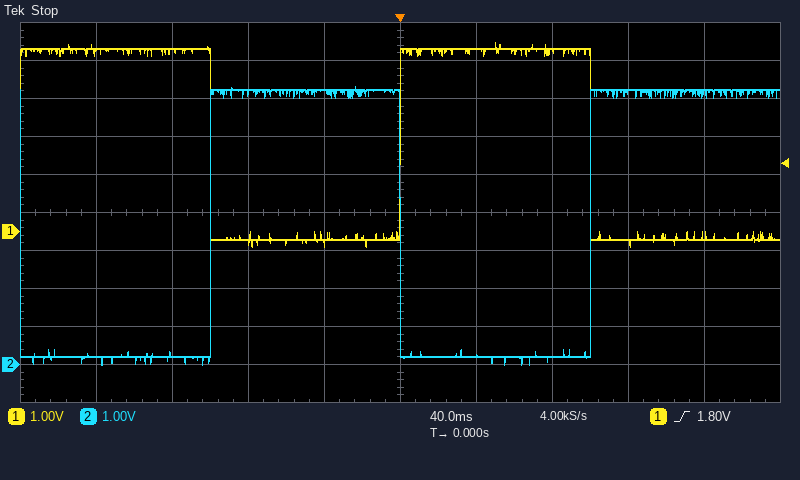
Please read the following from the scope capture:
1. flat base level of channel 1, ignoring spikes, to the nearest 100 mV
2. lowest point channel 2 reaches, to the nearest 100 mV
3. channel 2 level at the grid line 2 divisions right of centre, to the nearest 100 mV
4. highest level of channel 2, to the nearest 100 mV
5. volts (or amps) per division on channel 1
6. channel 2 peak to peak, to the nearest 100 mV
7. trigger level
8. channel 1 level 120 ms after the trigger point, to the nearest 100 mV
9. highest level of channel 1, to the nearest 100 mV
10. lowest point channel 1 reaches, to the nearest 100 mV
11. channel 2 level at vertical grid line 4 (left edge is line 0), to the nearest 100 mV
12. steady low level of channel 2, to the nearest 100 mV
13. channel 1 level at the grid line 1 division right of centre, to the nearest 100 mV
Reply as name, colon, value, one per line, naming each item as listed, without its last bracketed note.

flat base level of channel 1, ignoring spikes, to the nearest 100 mV: -200 mV
lowest point channel 2 reaches, to the nearest 100 mV: 0.0 V
channel 2 level at the grid line 2 divisions right of centre, to the nearest 100 mV: 200 mV
highest level of channel 2, to the nearest 100 mV: 7.3 V
volts (or amps) per division on channel 1: 1 V
channel 2 peak to peak, to the nearest 100 mV: 7.3 V
trigger level: 1.80 V
channel 1 level 120 ms after the trigger point, to the nearest 100 mV: -300 mV
highest level of channel 1, to the nearest 100 mV: 5.0 V
lowest point channel 1 reaches, to the nearest 100 mV: -400 mV
channel 2 level at vertical grid line 4 (left edge is line 0), to the nearest 100 mV: 7.2 V
steady low level of channel 2, to the nearest 100 mV: 200 mV
channel 1 level at the grid line 1 division right of centre, to the nearest 100 mV: 4.8 V
